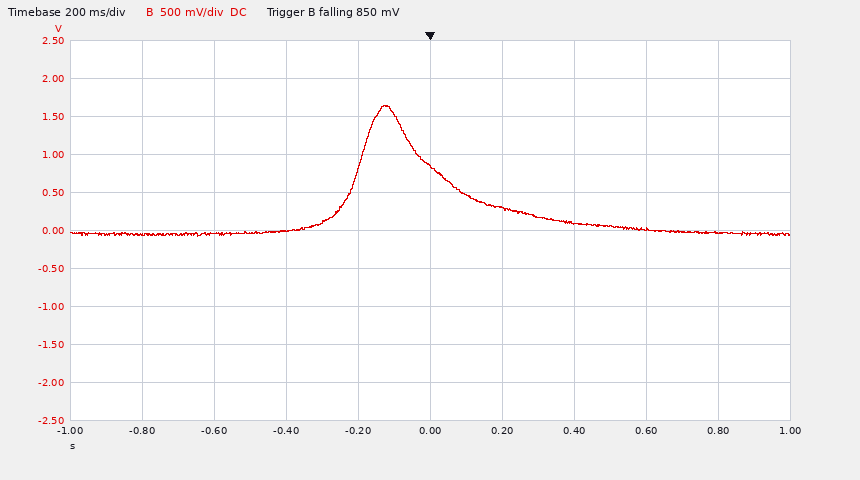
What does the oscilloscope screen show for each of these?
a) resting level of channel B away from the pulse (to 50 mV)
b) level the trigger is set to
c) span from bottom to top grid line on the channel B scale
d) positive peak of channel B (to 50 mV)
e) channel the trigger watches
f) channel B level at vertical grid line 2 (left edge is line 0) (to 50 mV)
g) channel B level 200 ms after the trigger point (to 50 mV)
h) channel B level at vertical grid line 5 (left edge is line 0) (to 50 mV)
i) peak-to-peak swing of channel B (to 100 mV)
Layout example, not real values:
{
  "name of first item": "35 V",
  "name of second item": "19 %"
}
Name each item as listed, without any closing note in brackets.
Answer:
{
  "resting level of channel B away from the pulse": "-50 mV",
  "level the trigger is set to": "850 mV",
  "span from bottom to top grid line on the channel B scale": "5 V",
  "positive peak of channel B": "1.65 V",
  "channel the trigger watches": "channel B",
  "channel B level at vertical grid line 2 (left edge is line 0)": "-50 mV",
  "channel B level 200 ms after the trigger point": "300 mV",
  "channel B level at vertical grid line 5 (left edge is line 0)": "850 mV",
  "peak-to-peak swing of channel B": "1.70 V"
}
